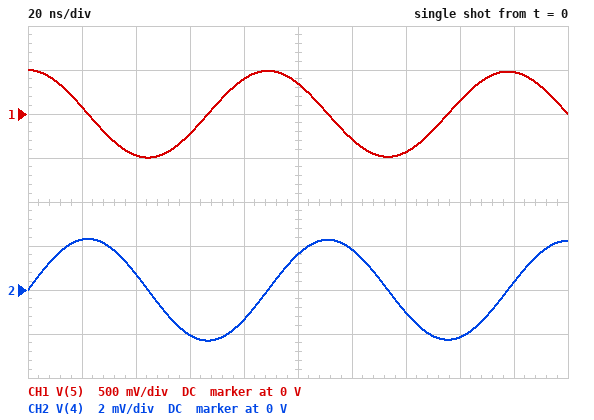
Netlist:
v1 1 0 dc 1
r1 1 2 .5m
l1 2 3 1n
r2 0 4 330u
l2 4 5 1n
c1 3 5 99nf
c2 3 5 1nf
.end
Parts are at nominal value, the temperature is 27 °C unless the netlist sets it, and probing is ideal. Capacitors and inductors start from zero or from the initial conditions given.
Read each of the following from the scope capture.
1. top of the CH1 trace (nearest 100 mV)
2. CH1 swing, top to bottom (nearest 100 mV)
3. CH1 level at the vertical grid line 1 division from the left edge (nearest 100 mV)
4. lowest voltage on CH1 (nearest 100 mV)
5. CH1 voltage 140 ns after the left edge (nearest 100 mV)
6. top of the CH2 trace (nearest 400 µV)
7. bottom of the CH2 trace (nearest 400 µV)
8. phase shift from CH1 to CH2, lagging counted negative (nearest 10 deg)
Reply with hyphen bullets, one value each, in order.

- 500 mV
- 1.0 V
- 100 mV
- -500 mV
- -400 mV
- 2.4 mV
- -2.4 mV
- -90 deg
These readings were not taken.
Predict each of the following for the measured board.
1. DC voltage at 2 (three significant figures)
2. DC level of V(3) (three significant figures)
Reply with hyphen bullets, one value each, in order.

- 1.00 V
- 1.00 V
